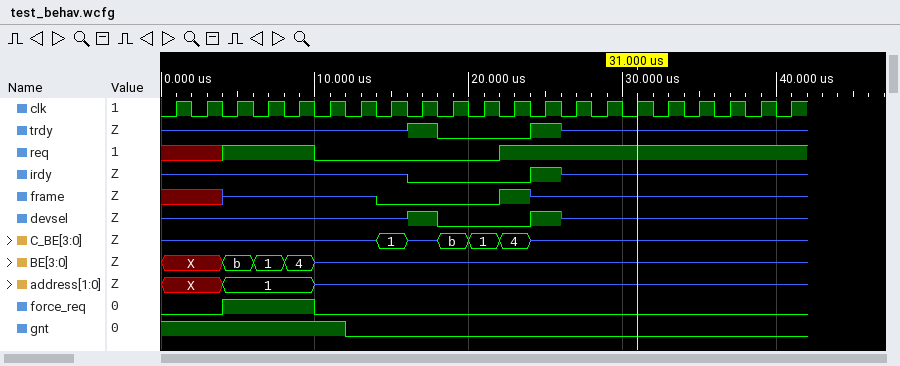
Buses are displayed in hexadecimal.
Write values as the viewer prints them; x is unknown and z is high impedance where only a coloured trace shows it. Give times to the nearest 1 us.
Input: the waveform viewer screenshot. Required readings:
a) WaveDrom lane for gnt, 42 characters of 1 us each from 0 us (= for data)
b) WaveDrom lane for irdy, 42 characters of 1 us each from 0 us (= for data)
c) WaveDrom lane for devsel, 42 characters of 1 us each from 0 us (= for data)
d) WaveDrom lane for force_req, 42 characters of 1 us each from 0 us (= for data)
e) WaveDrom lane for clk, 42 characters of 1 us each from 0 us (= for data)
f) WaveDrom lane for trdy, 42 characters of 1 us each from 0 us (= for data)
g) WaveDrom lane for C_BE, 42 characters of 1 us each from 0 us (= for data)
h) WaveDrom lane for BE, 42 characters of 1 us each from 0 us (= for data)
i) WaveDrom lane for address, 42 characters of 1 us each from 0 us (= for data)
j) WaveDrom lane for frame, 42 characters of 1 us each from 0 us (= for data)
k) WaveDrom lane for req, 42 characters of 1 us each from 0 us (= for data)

{name: 'gnt', wave: '1...........0.............................'}
{name: 'irdy', wave: 'z...............0.......1.z...............'}
{name: 'devsel', wave: 'z...............1.0.....1.z...............'}
{name: 'force_req', wave: '0...1.....0...............................'}
{name: 'clk', wave: '010101010101010101010101010101010101010101'}
{name: 'trdy', wave: 'z...............1.0.....1.z...............'}
{name: 'C_BE', wave: 'z.............=.z.=.=.=.z.................', data: '1 b 1 4'}
{name: 'BE', wave: 'x...=.=.=.z...............................', data: 'b 1 4'}
{name: 'address', wave: 'x...=.....z...............................', data: '1'}
{name: 'frame', wave: 'x...z.........0.......1.z.................'}
{name: 'req', wave: 'x...1.....0...........1...................'}
